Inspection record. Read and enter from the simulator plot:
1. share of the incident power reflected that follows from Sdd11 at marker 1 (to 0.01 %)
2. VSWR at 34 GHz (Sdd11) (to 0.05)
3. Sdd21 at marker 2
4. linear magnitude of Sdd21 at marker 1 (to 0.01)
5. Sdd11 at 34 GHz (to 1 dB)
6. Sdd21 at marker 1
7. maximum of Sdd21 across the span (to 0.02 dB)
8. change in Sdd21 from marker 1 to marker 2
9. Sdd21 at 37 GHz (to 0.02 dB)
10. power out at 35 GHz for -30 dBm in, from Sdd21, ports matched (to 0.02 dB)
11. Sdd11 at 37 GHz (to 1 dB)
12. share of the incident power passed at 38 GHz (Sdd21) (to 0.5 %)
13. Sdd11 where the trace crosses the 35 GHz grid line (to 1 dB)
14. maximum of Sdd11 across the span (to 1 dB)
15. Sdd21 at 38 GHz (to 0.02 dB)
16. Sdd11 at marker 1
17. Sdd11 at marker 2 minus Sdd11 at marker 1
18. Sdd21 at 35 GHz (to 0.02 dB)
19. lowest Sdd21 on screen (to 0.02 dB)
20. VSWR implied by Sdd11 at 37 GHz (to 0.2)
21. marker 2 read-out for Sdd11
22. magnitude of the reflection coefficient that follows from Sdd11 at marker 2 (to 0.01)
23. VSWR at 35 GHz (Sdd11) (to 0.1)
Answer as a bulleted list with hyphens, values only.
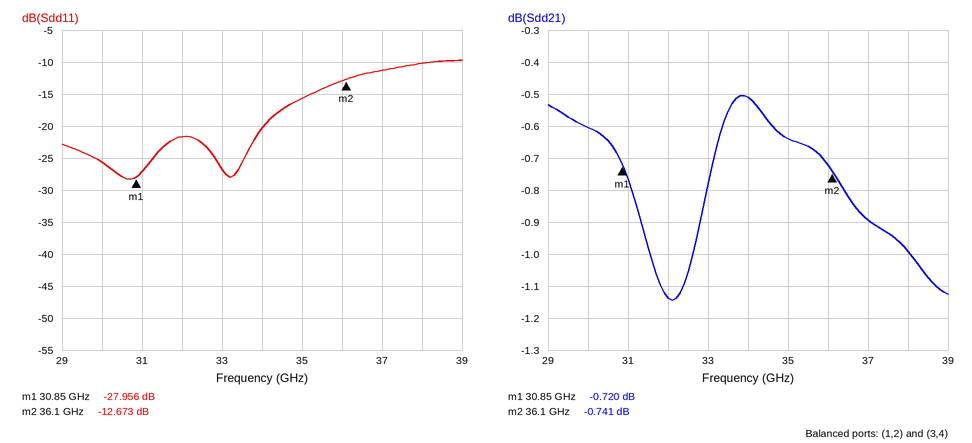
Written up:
- 0.16 %
- 1.20
- -0.741 dB
- 0.92
- -20 dB
- -0.720 dB
- -0.50 dB
- -0.021 dB
- -0.90 dB
- -30.64 dBm
- -11 dB
- 79.5 %
- -16 dB
- -10 dB
- -1.00 dB
- -27.956 dB
- 15.283 dB
- -0.64 dB
- -1.14 dB
- 1.8
- -12.673 dB
- 0.23
- 1.4
